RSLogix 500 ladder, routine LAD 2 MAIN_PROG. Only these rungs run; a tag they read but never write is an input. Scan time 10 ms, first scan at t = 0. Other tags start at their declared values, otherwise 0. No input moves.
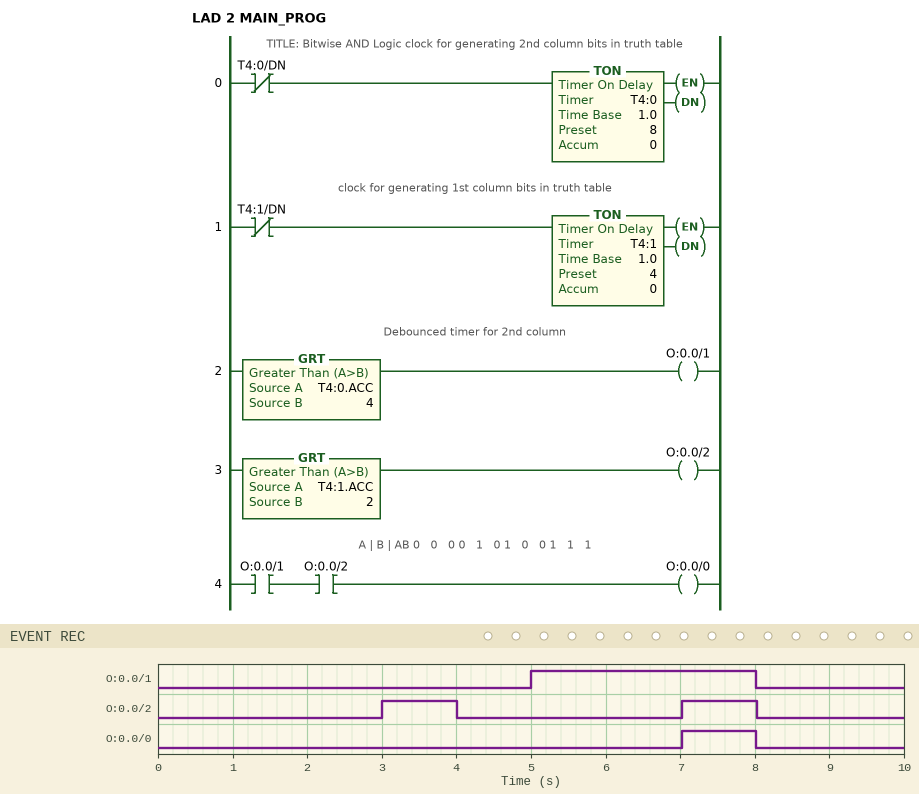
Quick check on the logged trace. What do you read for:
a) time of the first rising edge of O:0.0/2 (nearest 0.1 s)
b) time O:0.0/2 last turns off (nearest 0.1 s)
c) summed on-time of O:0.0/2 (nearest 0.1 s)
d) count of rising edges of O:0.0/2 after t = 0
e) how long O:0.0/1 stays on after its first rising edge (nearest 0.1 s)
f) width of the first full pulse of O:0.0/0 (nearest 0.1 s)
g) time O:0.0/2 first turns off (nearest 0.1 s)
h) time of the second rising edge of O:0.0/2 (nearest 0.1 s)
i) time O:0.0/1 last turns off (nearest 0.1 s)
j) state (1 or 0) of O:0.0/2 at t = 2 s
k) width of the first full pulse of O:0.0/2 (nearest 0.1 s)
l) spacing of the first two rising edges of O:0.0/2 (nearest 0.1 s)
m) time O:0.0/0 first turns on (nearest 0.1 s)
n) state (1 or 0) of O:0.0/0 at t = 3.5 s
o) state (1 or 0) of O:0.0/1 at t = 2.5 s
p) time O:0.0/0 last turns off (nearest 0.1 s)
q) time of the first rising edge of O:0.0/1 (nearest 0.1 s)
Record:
3.0 s
8.0 s
2.0 s
2
3.0 s
1.0 s
4.0 s
7.0 s
8.0 s
0
1.0 s
4.0 s
7.0 s
0
0
8.0 s
5.0 s
